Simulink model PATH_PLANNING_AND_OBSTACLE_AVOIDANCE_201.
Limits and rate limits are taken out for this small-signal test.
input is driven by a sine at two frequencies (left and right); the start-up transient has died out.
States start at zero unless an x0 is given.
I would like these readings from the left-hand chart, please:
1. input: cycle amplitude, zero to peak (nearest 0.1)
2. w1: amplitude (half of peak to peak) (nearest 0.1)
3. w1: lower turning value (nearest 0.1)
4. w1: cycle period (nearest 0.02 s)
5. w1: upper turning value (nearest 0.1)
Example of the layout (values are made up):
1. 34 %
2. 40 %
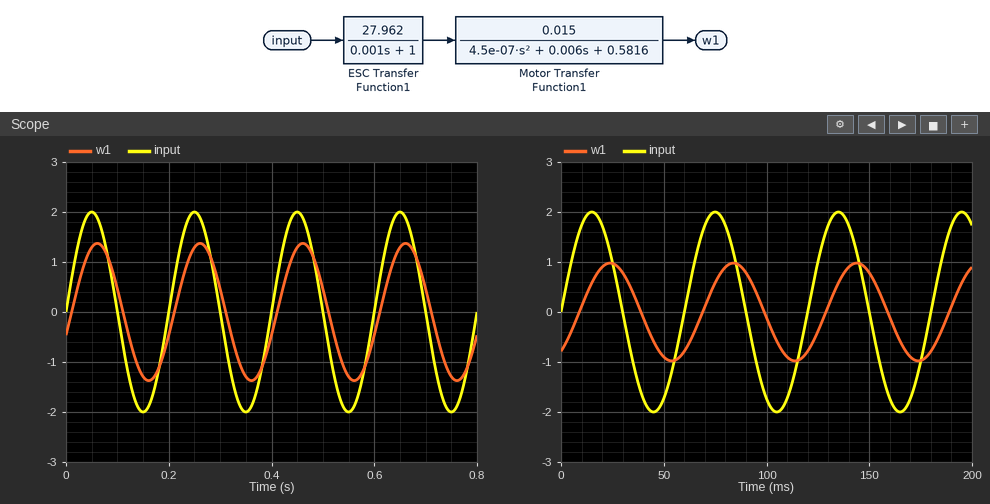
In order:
1. 2.0
2. 1.4
3. -1.4
4. 0.20 s
5. 1.4
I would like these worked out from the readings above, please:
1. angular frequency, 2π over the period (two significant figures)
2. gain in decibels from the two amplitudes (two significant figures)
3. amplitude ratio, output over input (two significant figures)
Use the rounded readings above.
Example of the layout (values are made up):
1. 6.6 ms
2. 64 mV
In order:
1. 31 rad/s
2. -3.1 dB
3. 0.70
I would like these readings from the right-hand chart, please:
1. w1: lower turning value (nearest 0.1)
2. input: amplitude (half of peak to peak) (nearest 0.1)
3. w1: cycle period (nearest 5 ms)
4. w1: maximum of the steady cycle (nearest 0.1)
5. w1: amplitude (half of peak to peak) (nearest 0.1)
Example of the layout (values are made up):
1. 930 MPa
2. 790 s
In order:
1. -1.0
2. 2.0
3. 60 ms
4. 1.0
5. 1.0
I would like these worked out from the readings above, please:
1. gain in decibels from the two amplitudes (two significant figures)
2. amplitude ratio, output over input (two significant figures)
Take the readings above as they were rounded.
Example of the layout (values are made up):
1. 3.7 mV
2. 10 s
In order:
1. -6.0 dB
2. 0.50
